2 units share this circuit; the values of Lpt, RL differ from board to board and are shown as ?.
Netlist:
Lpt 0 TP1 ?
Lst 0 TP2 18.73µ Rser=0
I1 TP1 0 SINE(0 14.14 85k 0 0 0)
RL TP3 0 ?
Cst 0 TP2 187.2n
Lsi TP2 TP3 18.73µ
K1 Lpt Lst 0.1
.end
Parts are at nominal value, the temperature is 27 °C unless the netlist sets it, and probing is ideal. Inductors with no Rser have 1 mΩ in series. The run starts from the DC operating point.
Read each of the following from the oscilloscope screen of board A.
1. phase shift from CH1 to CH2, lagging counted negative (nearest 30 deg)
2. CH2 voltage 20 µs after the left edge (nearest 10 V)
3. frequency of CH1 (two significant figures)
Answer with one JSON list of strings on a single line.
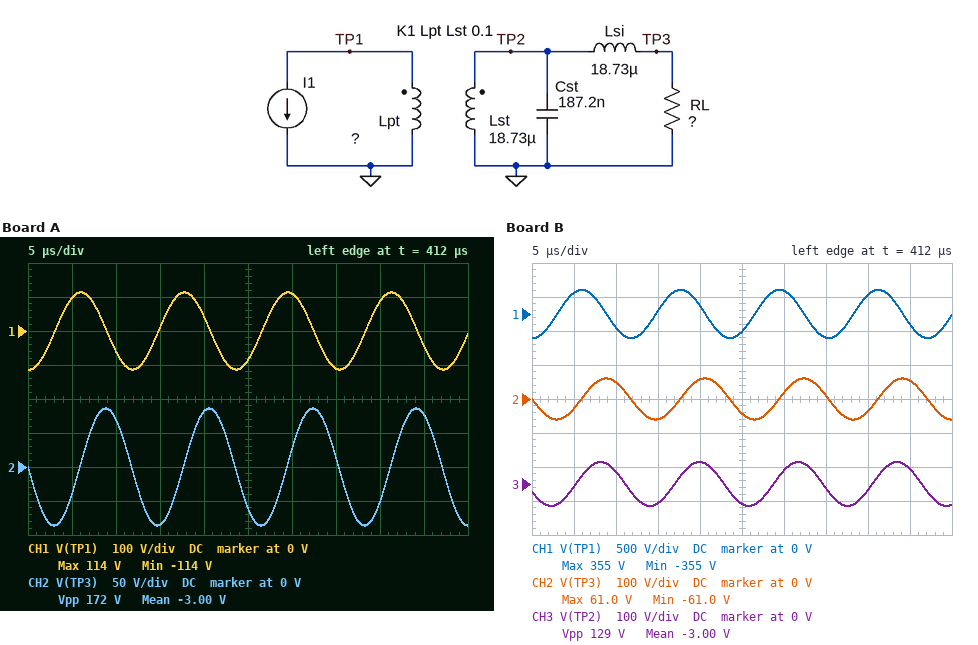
["-90 deg", "80 V", "85 kHz"]
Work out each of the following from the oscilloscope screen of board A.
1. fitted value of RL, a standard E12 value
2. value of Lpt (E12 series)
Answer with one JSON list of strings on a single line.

["68 Ω", "15 µH"]
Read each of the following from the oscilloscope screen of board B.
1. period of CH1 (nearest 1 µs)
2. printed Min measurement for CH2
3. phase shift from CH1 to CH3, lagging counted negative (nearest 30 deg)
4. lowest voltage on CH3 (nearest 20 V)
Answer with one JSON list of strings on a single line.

["12 µs", "-61.0 V", "-60 deg", "-60 V"]
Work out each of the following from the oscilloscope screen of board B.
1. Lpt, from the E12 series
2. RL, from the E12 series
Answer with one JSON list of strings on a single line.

["47 µH", "27 Ω"]
